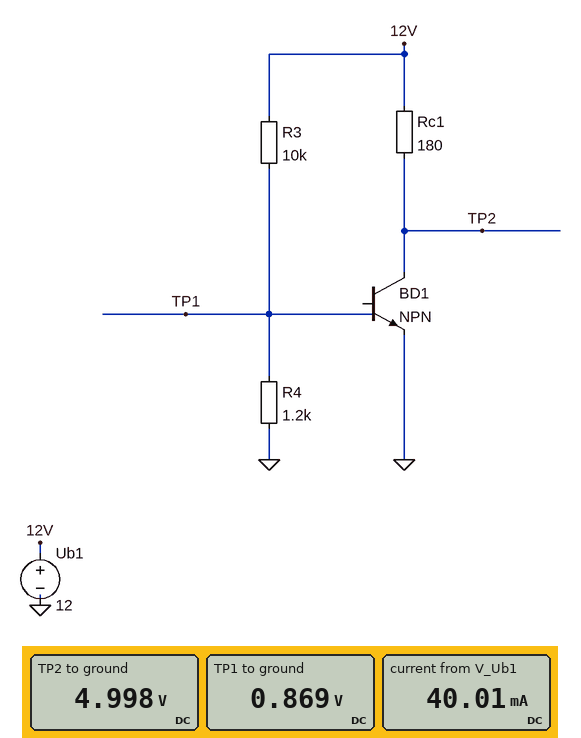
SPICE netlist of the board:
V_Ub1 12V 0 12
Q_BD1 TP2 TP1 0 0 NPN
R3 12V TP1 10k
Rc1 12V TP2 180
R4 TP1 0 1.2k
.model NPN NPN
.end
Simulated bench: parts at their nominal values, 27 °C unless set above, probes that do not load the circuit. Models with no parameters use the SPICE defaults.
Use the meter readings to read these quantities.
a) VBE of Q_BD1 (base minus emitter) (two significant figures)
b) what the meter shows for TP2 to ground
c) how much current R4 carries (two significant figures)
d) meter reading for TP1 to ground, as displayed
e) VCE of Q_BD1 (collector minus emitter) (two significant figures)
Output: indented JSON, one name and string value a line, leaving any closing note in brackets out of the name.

{
  "VBE of Q_BD1 (base minus emitter)": "870 mV",
  "what the meter shows for TP2 to ground": "4.998 V",
  "how much current R4 carries": "720 µA",
  "meter reading for TP1 to ground, as displayed": "0.869 V",
  "VCE of Q_BD1 (collector minus emitter)": "5.0 V"
}
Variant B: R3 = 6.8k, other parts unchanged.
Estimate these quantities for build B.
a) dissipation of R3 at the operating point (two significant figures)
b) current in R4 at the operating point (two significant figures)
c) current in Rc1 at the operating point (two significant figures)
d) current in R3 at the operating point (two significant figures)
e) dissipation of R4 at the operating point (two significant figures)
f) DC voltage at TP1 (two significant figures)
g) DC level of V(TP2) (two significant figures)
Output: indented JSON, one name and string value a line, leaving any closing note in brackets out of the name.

{
  "dissipation of R3 at the operating point": "18 mW",
  "current in R4 at the operating point": "740 µA",
  "current in Rc1 at the operating point": "66 mA",
  "current in R3 at the operating point": "1.6 mA",
  "dissipation of R4 at the operating point": "650 µW",
  "DC voltage at TP1": "880 mV",
  "DC level of V(TP2)": "150 mV"
}
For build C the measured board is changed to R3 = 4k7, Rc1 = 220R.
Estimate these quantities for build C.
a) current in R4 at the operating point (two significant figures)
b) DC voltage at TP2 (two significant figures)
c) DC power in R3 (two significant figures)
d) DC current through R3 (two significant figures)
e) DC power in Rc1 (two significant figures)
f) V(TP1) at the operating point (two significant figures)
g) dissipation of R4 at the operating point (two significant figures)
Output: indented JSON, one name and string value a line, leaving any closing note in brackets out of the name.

{
  "current in R4 at the operating point": "730 µA",
  "DC voltage at TP2": "100 mV",
  "DC power in R3": "26 mW",
  "DC current through R3": "2.4 mA",
  "DC power in Rc1": "640 mW",
  "V(TP1) at the operating point": "880 mV",
  "dissipation of R4 at the operating point": "640 µW"
}
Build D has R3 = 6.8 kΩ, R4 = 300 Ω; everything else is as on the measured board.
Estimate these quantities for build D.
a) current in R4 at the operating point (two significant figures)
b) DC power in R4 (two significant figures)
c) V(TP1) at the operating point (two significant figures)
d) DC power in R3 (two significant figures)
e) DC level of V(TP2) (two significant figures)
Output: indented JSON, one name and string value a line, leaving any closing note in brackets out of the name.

{
  "current in R4 at the operating point": "1.7 mA",
  "DC power in R4": "860 µW",
  "V(TP1) at the operating point": "510 mV",
  "DC power in R3": "19 mW",
  "DC level of V(TP2)": "12 V"
}
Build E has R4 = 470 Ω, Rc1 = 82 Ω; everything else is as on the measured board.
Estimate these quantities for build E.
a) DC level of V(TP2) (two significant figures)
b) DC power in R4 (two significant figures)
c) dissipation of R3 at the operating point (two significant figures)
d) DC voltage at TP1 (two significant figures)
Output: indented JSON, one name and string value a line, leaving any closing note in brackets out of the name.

{
  "DC level of V(TP2)": "12 V",
  "DC power in R4": "620 µW",
  "dissipation of R3 at the operating point": "13 mW",
  "DC voltage at TP1": "540 mV"
}
